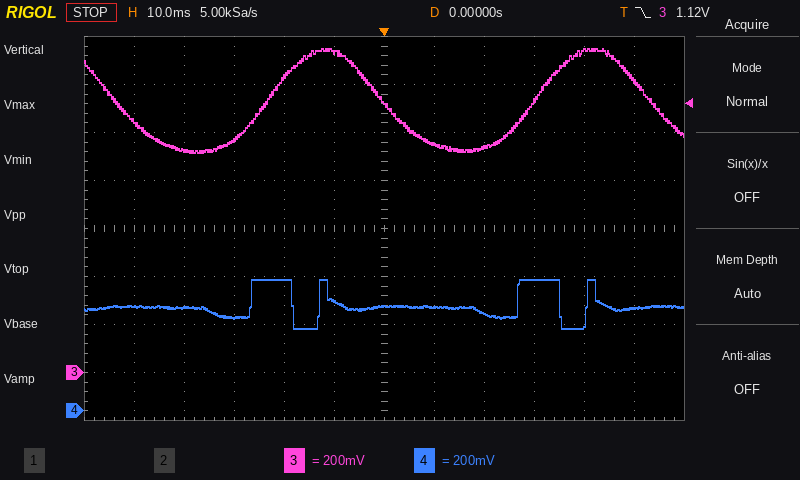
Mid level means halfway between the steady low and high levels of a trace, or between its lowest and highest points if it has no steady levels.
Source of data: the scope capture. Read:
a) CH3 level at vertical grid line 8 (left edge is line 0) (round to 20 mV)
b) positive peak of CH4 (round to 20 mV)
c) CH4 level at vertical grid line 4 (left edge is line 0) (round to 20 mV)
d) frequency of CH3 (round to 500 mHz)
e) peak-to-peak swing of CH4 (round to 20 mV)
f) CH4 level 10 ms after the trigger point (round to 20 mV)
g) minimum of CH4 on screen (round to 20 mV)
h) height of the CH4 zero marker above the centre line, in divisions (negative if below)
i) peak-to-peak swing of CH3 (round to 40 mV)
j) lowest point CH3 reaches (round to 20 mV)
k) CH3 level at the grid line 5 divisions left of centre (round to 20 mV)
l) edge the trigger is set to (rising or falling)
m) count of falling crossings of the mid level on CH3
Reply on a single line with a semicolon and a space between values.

940 mV; 540 mV; 540 mV; 18.5 Hz; 200 mV; 440 mV; 340 mV; -3.8 div; 440 mV; 920 mV; 1.04 V; falling; 3
